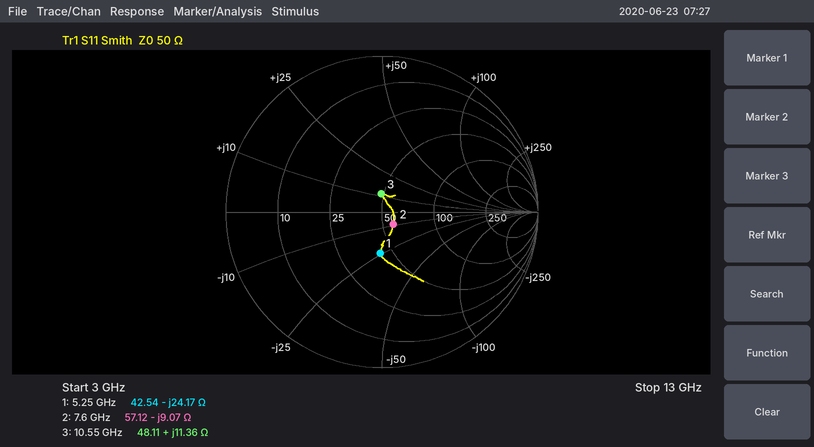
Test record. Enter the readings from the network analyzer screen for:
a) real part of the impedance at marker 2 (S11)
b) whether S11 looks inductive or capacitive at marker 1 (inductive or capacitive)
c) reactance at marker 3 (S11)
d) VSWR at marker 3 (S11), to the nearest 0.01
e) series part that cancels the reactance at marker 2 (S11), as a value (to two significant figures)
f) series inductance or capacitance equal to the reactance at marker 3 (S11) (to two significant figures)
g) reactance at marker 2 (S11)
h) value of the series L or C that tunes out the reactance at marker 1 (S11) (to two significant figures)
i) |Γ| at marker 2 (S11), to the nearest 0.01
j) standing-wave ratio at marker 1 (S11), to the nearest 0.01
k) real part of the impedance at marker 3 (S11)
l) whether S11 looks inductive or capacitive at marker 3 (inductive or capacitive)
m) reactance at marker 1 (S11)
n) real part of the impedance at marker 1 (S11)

57.12 Ω
capacitive
+11.36 Ω
1.26
190 pH
170 pH
-9.07 Ω
730 pH
0.11
1.72
48.11 Ω
inductive
-24.17 Ω
42.54 Ω
